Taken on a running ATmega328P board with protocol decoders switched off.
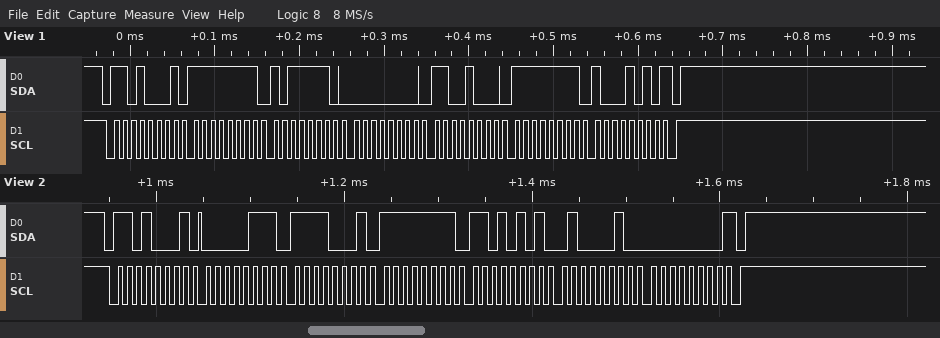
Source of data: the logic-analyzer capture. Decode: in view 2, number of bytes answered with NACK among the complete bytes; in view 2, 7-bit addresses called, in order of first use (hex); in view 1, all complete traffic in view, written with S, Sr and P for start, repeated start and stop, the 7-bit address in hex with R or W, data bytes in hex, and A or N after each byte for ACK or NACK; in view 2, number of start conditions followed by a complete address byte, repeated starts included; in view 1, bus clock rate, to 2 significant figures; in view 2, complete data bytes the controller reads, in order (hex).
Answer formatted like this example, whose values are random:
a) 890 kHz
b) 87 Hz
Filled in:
a) 1
b) 0x68
c) S 68R A FF A BE A 00 A C8 A FF A 8A N P
d) 1
e) 100 kHz
f) 07 F1 FF D5 42 00
